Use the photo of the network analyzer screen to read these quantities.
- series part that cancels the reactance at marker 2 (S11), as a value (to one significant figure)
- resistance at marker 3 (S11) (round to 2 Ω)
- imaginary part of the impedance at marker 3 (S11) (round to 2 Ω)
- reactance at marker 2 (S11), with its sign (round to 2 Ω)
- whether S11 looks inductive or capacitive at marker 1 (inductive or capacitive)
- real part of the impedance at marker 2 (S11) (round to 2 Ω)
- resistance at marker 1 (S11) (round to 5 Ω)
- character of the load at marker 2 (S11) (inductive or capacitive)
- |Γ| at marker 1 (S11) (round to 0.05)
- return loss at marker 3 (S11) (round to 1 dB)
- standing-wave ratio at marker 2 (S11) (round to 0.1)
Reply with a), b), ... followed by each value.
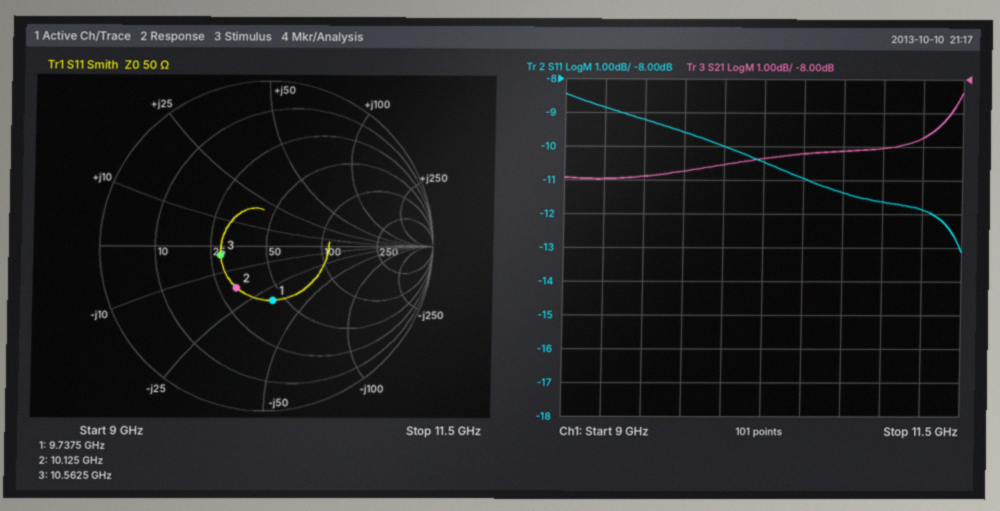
a) 300 pH
b) 28 Ω
c) -4 Ω
d) -18 Ω
e) capacitive
f) 32 Ω
g) 45 Ω
h) capacitive
i) 0.35
j) 11 dB
k) 1.9
